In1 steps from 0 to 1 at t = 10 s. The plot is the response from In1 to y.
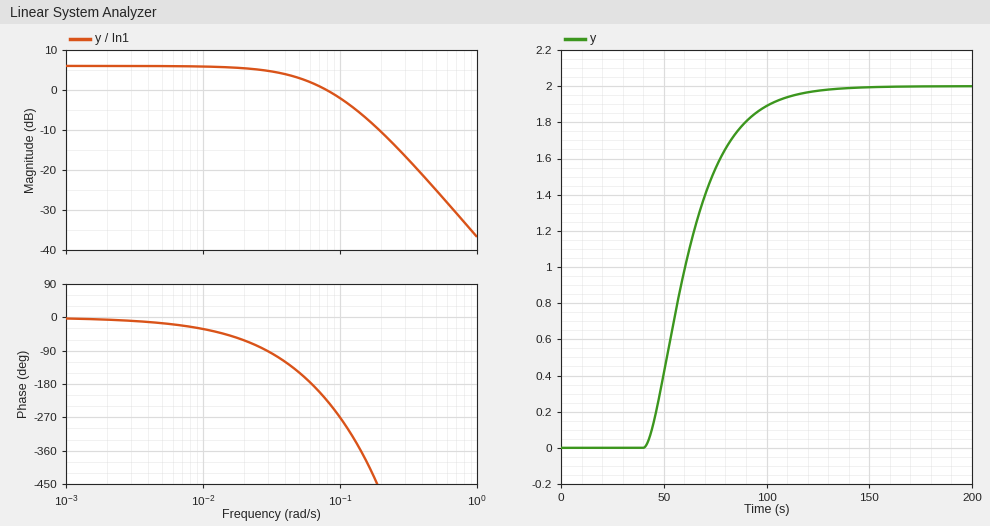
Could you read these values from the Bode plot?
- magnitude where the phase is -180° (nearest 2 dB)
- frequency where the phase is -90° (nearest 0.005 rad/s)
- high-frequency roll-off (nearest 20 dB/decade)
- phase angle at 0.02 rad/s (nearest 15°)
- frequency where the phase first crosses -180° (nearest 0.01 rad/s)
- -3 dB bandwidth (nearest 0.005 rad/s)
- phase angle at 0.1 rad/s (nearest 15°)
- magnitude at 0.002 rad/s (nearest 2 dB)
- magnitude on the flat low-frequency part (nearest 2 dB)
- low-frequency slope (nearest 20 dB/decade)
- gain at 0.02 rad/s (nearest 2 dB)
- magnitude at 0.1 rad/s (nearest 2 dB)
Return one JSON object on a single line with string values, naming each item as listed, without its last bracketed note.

{"magnitude where the phase is -180°": "2 dB", "frequency where the phase is -90°": "0.030 rad/s", "high-frequency roll-off": "-40 dB/decade", "phase angle at 0.02 rad/s": "-60°", "frequency where the phase first crosses -180°": "0.06 rad/s", "-3 dB bandwidth": "0.050 rad/s", "phase angle at 0.1 rad/s": "-270°", "magnitude at 0.002 rad/s": "6 dB", "magnitude on the flat low-frequency part": "6 dB", "low-frequency slope": "0 dB/decade", "gain at 0.02 rad/s": "6 dB", "magnitude at 0.1 rad/s": "-2 dB"}
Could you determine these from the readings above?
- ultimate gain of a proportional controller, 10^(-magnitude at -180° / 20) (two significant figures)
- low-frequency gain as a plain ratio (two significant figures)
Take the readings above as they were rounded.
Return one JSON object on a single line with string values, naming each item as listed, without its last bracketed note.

{"ultimate gain of a proportional controller, 10^(-magnitude at -180° / 20)": "0.79", "low-frequency gain as a plain ratio": "2.0"}
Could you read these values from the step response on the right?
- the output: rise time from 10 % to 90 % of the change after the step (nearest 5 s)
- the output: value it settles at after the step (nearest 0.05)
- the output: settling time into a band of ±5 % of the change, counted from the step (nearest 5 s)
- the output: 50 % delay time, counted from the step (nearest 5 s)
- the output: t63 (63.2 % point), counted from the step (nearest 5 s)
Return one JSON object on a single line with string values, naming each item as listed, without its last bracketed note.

{"the output: rise time from 10 % to 90 % of the change after the step": "45 s", "the output: value it settles at after the step": "2.00", "the output: settling time into a band of ±5 % of the change, counted from the step": "90 s", "the output: 50 % delay time, counted from the step": "50 s", "the output: t63 (63.2 % point), counted from the step": "55 s"}
